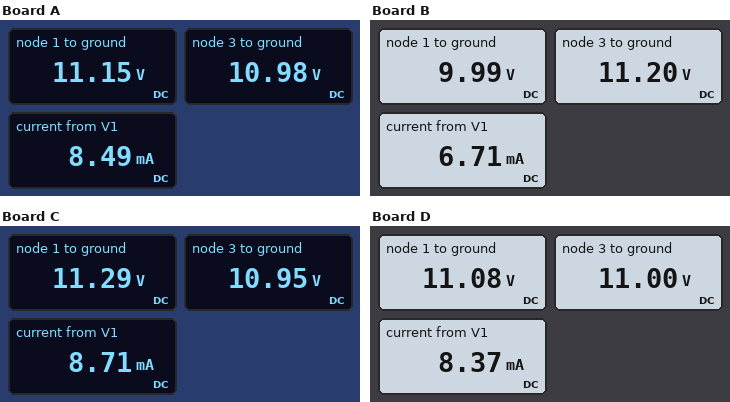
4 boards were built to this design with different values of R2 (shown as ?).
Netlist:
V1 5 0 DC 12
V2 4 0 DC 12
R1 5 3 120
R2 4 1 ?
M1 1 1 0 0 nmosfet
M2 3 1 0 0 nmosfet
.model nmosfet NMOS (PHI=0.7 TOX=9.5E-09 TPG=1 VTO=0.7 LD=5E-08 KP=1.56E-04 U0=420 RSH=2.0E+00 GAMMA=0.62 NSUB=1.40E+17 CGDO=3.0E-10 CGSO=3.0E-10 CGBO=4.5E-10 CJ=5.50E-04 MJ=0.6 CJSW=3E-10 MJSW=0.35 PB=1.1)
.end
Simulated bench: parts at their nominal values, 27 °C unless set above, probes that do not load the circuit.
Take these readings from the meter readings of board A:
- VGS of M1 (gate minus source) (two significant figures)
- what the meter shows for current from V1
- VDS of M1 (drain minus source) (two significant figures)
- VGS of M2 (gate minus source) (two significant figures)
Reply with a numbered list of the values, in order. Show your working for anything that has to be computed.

1. 11.15 V = 11 V
2. 8.49 mA
3. 11.15 V = 11 V
4. 11.15 V = 11 V
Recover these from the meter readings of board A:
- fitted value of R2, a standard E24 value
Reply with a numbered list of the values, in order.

1. 100 Ω
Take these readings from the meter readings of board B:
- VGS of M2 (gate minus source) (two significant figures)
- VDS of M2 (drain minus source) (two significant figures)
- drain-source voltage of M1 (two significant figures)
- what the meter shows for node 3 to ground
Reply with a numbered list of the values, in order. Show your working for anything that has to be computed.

1. 9.99 V = 10 V
2. 11.2 V = 11 V
3. 9.99 V = 10 V
4. 11.20 V
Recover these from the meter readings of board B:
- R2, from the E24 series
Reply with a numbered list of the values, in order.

1. 300 Ω
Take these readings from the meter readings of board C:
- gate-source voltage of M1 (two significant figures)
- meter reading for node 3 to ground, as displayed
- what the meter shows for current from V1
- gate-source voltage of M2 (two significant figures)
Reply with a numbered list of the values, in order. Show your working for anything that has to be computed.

1. 11.29 V = 11 V
2. 10.95 V
3. 8.71 mA
4. 11.29 V = 11 V
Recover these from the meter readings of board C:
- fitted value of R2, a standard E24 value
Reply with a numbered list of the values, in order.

1. 82 Ω
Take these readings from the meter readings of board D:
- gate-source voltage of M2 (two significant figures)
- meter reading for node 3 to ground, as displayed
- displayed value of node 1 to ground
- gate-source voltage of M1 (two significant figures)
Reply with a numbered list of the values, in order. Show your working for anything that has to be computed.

1. 11.08 V = 11 V
2. 11.00 V
3. 11.08 V
4. 11.08 V = 11 V
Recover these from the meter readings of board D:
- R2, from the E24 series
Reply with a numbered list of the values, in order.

1. 110 Ω
